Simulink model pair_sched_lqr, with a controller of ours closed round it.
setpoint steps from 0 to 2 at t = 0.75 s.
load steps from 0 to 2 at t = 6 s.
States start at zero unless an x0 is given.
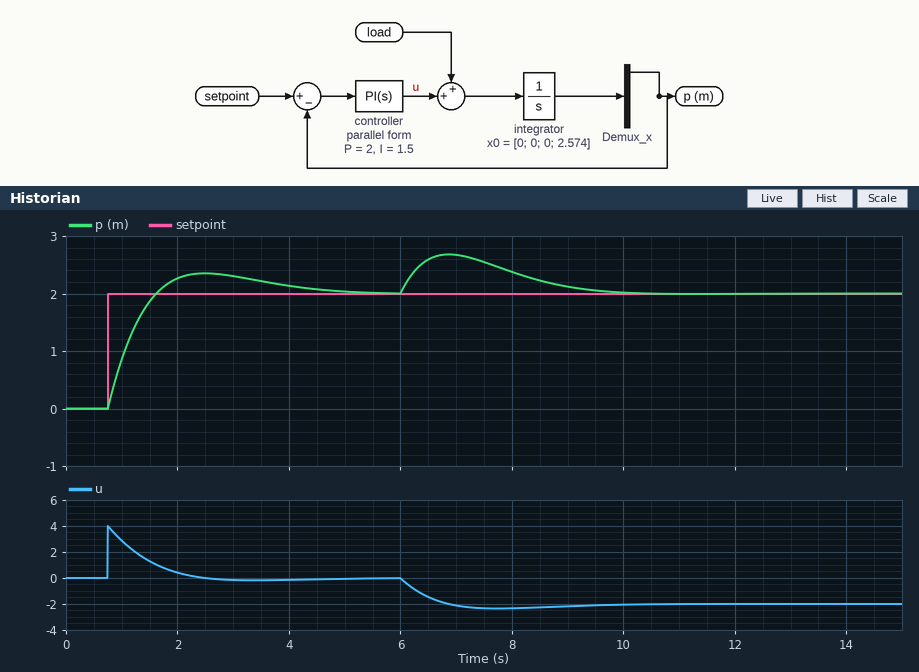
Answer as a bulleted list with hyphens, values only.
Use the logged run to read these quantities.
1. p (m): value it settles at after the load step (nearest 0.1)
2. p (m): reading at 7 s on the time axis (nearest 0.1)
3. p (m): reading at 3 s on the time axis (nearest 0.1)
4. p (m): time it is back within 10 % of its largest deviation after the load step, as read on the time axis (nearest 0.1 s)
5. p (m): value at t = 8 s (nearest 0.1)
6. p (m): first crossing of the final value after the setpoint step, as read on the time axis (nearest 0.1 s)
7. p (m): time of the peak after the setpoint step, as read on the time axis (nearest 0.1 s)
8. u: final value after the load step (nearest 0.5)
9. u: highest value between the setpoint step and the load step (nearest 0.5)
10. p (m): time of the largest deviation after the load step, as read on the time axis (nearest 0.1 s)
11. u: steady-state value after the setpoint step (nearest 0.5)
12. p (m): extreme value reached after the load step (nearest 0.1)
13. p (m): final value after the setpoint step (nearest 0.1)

- 2.0
- 2.7
- 2.3
- 9.4 s
- 2.4
- 1.6 s
- 2.5 s
- -2.0
- 4.0
- 6.9 s
- 0.0
- 2.7
- 2.0
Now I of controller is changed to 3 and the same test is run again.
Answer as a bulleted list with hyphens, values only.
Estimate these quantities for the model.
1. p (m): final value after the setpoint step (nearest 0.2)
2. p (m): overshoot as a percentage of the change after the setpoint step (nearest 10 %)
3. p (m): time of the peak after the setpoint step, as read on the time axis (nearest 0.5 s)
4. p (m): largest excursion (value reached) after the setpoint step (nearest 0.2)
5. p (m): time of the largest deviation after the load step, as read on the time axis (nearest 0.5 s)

- 2.0
- 30 %
- 2.0 s
- 2.6
- 6.5 s
